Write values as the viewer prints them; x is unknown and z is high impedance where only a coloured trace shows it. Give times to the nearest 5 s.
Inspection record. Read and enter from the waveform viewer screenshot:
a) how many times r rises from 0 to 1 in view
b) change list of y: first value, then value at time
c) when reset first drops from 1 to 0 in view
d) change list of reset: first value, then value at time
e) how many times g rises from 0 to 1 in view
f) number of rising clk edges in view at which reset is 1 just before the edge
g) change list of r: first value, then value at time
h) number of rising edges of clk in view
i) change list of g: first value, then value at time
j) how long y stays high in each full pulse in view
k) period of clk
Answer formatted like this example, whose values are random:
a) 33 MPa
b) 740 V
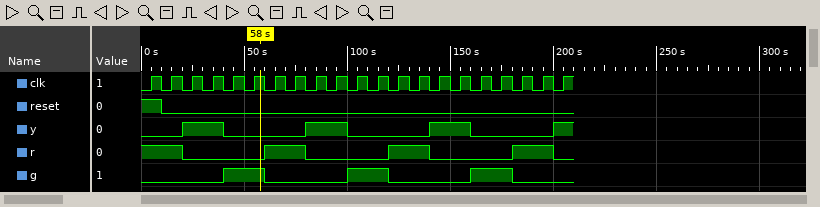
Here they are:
a) 3
b) 0, 1 at 20 s, 0 at 40 s, 1 at 80 s, 0 at 100 s, 1 at 140 s, 0 at 160 s, 1 at 200 s
c) 10 s
d) 1, 0 at 10 s
e) 3
f) 1
g) 1, 0 at 20 s, 1 at 60 s, 0 at 80 s, 1 at 120 s, 0 at 140 s, 1 at 180 s, 0 at 200 s
h) 21
i) 0, 1 at 40 s, 0 at 60 s, 1 at 100 s, 0 at 120 s, 1 at 160 s, 0 at 180 s
j) 20 s, 20 s, 20 s
k) 10 s
